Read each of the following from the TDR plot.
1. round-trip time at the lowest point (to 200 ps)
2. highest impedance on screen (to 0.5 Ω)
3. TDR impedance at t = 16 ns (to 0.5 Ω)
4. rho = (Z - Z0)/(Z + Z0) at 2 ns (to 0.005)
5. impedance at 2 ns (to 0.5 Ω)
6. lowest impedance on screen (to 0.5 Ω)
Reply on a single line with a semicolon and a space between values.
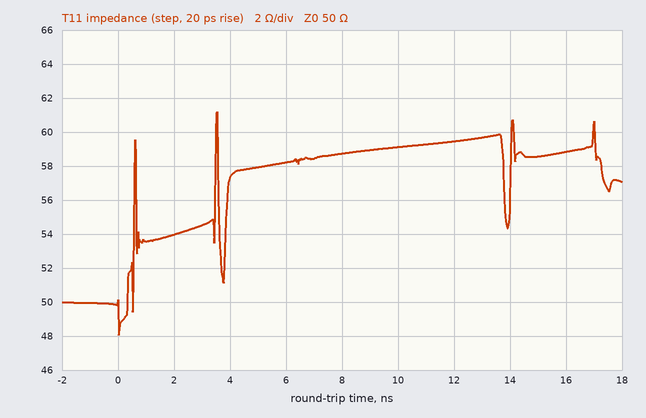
0.0 ns; 61.0 Ω; 59.0 Ω; +0.040; 54.0 Ω; 48.0 Ω
